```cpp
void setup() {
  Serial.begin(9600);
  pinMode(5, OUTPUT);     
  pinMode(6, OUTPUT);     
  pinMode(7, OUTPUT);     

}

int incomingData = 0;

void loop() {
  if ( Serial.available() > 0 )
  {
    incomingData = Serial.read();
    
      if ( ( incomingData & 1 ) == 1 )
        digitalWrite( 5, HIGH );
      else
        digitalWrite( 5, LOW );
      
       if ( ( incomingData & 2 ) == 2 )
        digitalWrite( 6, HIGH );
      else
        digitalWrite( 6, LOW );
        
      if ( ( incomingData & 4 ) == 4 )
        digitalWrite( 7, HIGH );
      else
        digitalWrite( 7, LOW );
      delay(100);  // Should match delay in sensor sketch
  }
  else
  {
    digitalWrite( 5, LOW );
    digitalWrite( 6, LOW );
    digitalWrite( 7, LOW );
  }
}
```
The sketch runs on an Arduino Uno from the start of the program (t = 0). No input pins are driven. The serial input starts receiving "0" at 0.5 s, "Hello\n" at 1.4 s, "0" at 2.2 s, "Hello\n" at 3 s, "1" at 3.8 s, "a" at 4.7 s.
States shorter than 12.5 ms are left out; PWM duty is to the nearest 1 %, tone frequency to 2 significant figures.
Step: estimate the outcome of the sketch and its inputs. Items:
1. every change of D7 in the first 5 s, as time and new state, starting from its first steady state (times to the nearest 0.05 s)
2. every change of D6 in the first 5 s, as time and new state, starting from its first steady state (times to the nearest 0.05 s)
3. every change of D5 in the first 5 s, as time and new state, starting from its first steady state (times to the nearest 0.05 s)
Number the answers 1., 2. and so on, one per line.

1. 0 s low; 1.5 s high; 1.9 s low; 3.1 s high; 3.5 s low
2. 0 s low; 1.8 s high; 2 s low; 3.4 s high; 3.6 s low
3. 0 s low; 1.5 s high; 1.6 s low; 1.8 s high; 1.9 s low; 3.1 s high; 3.2 s low; 3.4 s high; 3.5 s low; 3.8 s high; 3.9 s low; 4.7 s high; 4.8 s low
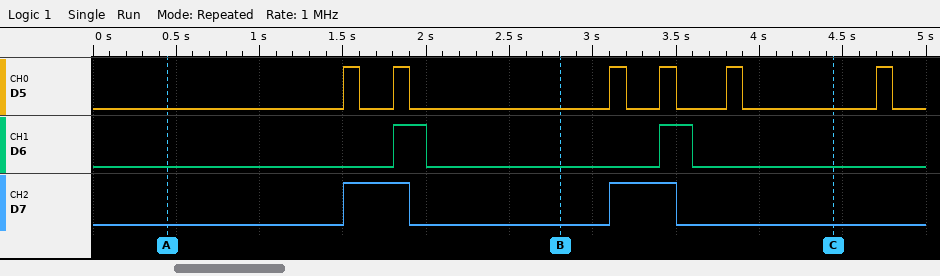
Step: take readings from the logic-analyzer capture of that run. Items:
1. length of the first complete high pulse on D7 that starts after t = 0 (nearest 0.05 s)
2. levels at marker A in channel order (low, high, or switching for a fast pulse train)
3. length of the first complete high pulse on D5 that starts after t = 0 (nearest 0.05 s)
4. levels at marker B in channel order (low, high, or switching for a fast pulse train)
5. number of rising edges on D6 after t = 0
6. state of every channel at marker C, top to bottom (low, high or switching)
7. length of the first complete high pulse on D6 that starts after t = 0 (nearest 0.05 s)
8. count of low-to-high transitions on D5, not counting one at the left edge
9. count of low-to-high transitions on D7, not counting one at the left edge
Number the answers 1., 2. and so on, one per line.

1. 0.40 s
2. D5 low, D6 low, D7 low
3. 0.10 s
4. D5 low, D6 low, D7 low
5. 2
6. D5 low, D6 low, D7 low
7. 0.20 s
8. 6
9. 2
